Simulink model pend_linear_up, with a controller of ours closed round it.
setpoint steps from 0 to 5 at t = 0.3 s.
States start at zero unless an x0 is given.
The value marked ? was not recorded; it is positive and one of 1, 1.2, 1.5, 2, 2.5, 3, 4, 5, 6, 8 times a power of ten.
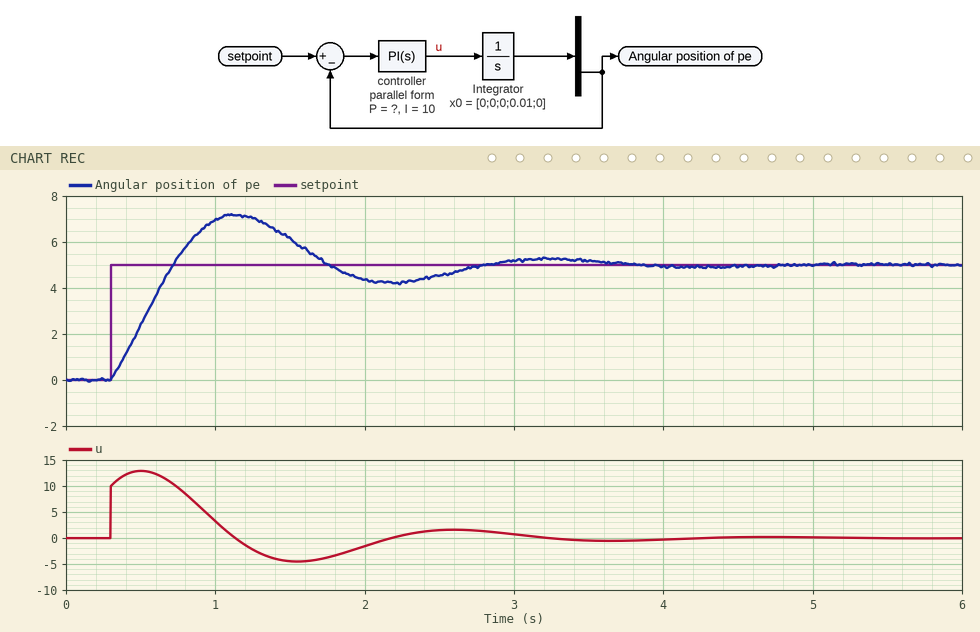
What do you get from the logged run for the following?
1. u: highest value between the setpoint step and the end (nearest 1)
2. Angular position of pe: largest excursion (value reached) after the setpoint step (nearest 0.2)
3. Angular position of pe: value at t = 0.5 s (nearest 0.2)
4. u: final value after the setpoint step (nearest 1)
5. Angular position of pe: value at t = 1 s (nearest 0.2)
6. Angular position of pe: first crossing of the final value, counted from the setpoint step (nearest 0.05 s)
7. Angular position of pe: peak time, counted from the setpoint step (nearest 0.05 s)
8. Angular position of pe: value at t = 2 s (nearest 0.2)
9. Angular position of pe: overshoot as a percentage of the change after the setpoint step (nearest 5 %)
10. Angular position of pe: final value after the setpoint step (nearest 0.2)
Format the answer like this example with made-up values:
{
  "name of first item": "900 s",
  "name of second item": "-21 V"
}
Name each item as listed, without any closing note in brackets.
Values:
{
  "u: highest value between the setpoint step and the end": "13",
  "Angular position of pe: largest excursion (value reached) after the setpoint step": "7.2",
  "Angular position of pe: value at t = 0.5 s": "2.4",
  "u: final value after the setpoint step": "0",
  "Angular position of pe: value at t = 1 s": "7.0",
  "Angular position of pe: first crossing of the final value, counted from the setpoint step": "0.40 s",
  "Angular position of pe: peak time, counted from the setpoint step": "0.85 s",
  "Angular position of pe: value at t = 2 s": "4.4",
  "Angular position of pe: overshoot as a percentage of the change after the setpoint step": "45 %",
  "Angular position of pe: final value after the setpoint step": "5.0"
}
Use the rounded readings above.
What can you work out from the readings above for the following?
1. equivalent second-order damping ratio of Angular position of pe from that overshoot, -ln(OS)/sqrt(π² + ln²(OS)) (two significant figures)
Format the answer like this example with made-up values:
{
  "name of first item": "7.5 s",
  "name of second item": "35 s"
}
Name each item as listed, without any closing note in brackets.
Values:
{
  "equivalent second-order damping ratio of Angular position of pe from that overshoot, -ln(OS)/sqrt(π² + ln²(OS))": "0.25"
}
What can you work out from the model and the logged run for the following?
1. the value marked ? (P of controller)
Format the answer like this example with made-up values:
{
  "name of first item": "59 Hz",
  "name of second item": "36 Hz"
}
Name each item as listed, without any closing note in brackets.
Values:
{
  "the value marked ?": "2"
}
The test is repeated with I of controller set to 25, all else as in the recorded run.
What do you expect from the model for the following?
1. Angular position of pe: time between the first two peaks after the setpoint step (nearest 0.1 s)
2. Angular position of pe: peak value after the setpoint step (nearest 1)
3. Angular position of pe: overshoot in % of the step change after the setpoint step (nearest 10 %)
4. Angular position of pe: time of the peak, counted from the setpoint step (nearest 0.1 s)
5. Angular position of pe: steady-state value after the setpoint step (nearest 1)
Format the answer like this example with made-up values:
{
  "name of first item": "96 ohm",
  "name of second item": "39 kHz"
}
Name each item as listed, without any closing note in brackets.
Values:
{
  "Angular position of pe: time between the first two peaks after the setpoint step": "1.3 s",
  "Angular position of pe: peak value after the setpoint step": "8",
  "Angular position of pe: overshoot in % of the step change after the setpoint step": "60 %",
  "Angular position of pe: time of the peak, counted from the setpoint step": "0.6 s",
  "Angular position of pe: steady-state value after the setpoint step": "5"
}
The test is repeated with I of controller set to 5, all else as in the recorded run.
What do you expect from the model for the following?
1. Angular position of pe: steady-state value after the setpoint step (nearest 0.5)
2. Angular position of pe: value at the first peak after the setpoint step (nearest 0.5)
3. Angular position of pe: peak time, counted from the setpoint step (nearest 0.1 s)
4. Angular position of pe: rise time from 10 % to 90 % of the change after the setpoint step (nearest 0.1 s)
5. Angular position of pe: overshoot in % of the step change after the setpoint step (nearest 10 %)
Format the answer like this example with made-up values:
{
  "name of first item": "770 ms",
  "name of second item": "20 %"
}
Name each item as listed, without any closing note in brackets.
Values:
{
  "Angular position of pe: steady-state value after the setpoint step": "5.0",
  "Angular position of pe: value at the first peak after the setpoint step": "6.5",
  "Angular position of pe: peak time, counted from the setpoint step": "1.1 s",
  "Angular position of pe: rise time from 10 % to 90 % of the change after the setpoint step": "0.4 s",
  "Angular position of pe: overshoot in % of the step change after the setpoint step": "30 %"
}
